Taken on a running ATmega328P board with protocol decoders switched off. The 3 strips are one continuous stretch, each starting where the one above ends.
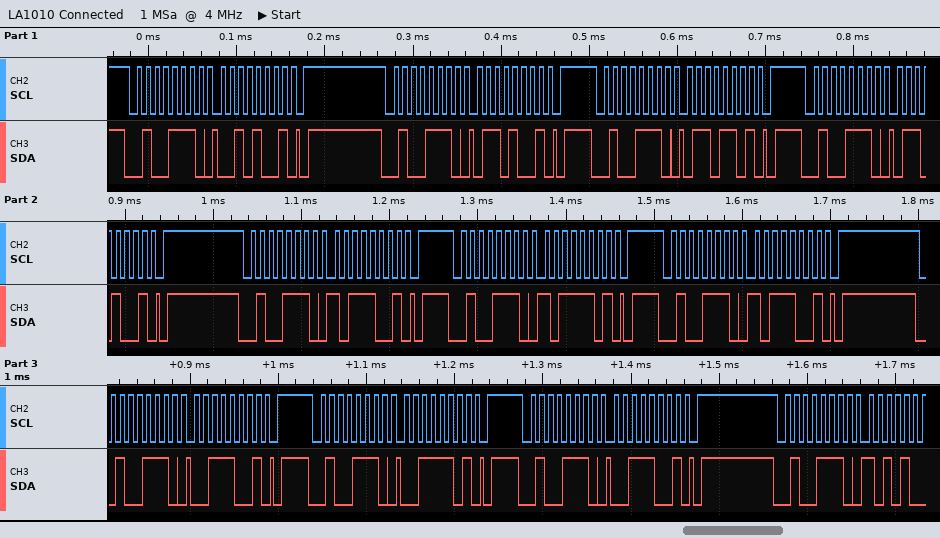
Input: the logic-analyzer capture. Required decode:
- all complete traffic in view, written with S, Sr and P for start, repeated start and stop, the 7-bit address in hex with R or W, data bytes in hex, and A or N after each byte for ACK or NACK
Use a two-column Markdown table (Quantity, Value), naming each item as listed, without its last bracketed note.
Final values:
| Quantity | Value |
|---|---|
| all complete traffic in view, written with S, Sr and P for start, repeated start and stop, the 7-bit address in hex with R or W, data bytes in hex, and A or N after each byte for ACK or NACK | S 27W A 29 A P S 27W A 69 A P S 27W A 6D A P S 27W A 69 A P S 27W A B9 A P S 27W A BD A P S 27W A B9 A P S 27W A 39 A P S 27W A 3D A P S 27W A 39 A P S 27W A |
